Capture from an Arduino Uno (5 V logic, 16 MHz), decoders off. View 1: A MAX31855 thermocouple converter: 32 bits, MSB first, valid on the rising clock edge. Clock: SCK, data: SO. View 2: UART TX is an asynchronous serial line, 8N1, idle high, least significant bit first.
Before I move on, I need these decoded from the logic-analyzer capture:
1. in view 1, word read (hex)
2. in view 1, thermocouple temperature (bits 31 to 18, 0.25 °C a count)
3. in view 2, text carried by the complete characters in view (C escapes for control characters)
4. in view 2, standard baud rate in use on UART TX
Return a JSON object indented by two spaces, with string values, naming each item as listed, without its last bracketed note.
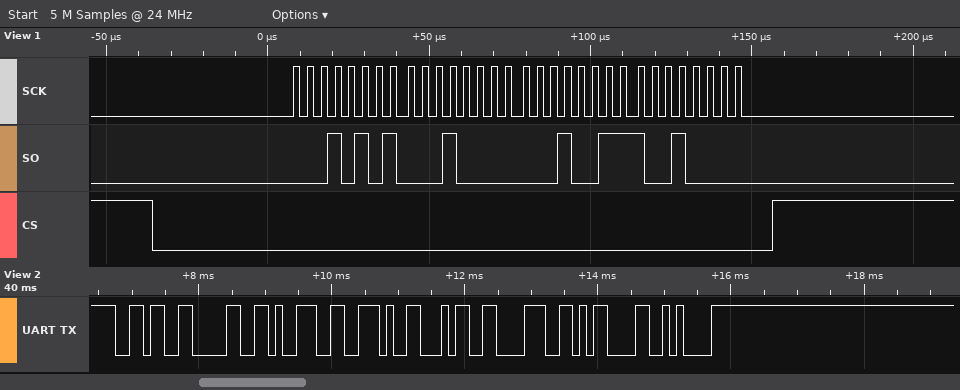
{
  "in view 1, word read": "0x15101390",
  "in view 1, thermocouple temperature": "337.00 °C",
  "in view 2, text carried by the complete characters in view": "\"609.48\\r\\n\"",
  "in view 2, standard baud rate in use on UART TX": "9600 baud"
}
